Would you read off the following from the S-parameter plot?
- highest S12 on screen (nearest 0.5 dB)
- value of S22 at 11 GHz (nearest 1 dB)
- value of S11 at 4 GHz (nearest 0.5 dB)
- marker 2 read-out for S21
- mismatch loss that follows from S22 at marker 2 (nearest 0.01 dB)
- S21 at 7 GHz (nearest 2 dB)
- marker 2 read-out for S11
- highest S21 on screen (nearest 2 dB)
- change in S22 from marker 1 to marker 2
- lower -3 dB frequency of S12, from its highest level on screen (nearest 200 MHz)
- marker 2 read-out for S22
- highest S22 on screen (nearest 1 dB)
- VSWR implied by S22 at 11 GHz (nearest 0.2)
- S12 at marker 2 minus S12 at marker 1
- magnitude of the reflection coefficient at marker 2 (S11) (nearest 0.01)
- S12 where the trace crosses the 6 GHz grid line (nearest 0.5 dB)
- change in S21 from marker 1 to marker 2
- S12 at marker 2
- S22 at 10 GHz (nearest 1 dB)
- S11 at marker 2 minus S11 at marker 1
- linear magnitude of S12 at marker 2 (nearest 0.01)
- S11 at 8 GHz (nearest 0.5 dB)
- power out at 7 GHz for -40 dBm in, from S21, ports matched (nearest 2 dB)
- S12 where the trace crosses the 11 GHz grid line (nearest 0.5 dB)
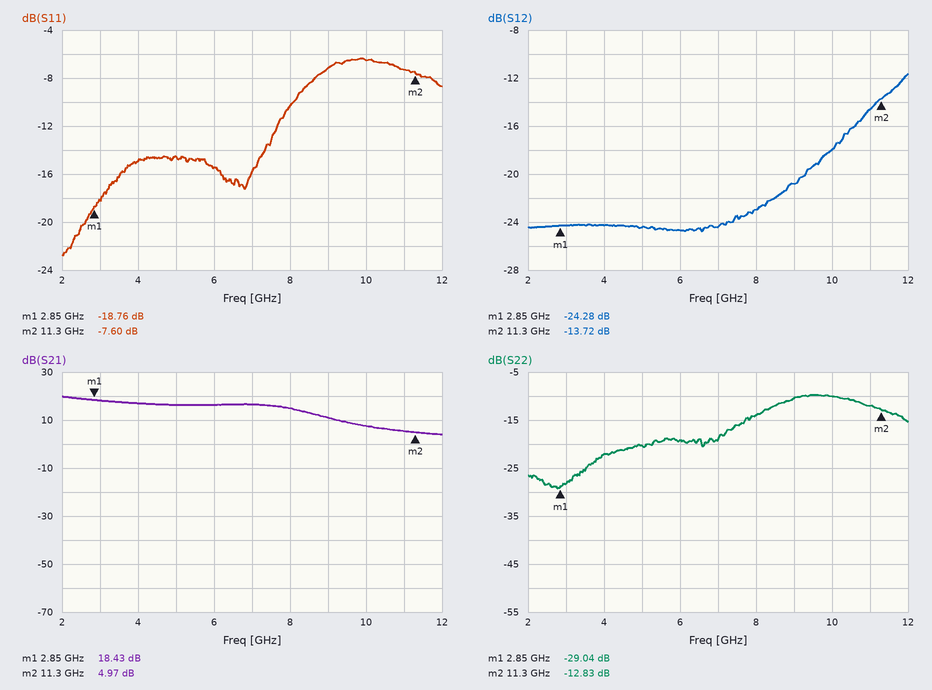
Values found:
-11.5 dB
-12 dB
-15.0 dB
4.97 dB
0.23 dB
16 dB
-7.60 dB
20 dB
16.21 dB
11.0 GHz
-12.83 dB
-10 dB
1.6
10.56 dB
0.42
-24.5 dB
-13.46 dB
-13.72 dB
-10 dB
11.16 dB
0.21
-10.5 dB
-24 dBm
-14.5 dB
